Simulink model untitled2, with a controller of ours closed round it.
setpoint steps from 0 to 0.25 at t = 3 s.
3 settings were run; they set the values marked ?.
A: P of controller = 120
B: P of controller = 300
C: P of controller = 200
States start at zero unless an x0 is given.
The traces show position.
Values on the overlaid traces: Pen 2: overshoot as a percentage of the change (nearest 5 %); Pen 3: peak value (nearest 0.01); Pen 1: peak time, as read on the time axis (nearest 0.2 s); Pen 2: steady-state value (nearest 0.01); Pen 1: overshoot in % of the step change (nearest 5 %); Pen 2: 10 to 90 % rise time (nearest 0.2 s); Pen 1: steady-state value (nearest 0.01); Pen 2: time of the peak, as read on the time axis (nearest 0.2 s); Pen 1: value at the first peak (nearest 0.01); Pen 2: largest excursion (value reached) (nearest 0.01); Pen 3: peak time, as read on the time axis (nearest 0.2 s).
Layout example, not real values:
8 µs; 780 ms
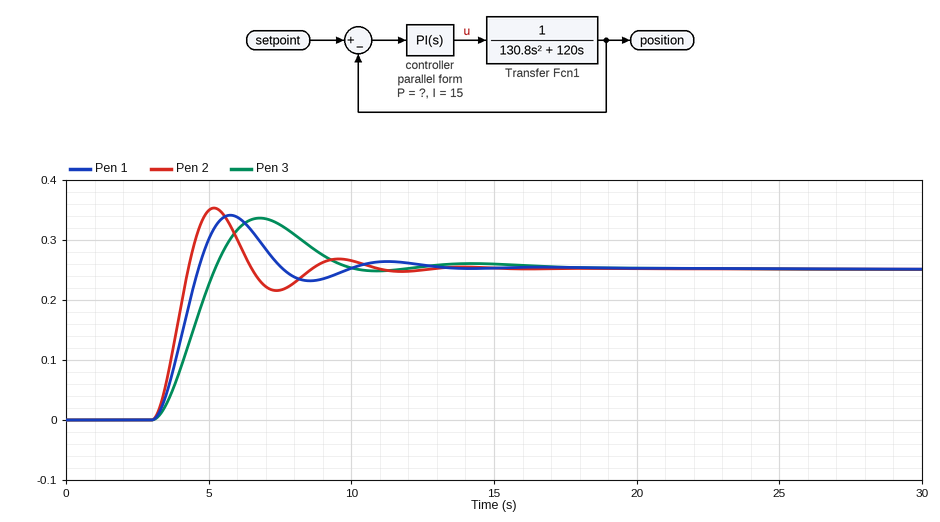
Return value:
40 %; 0.34; 5.8 s; 0.25; 35 %; 0.8 s; 0.25; 5.2 s; 0.34; 0.35; 6.8 s
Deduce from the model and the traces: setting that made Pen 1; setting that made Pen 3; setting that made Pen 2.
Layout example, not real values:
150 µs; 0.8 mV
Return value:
C; A; B
